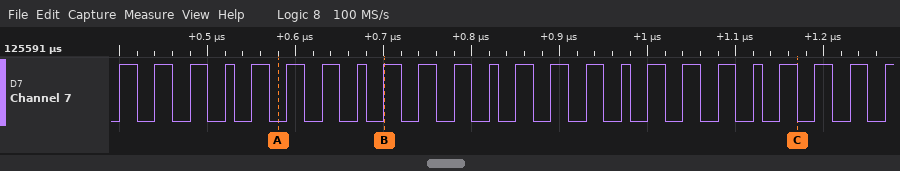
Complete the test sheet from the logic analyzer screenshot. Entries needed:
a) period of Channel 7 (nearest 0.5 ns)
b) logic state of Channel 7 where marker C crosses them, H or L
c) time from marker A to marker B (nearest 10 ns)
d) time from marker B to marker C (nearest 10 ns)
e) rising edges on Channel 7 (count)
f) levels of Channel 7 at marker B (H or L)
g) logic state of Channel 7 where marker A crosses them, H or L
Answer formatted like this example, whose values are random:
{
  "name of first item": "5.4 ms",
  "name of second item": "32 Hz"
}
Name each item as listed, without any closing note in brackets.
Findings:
{
  "period of Channel 7": "38 ns",
  "logic state of Channel 7 where marker C crosses them, H or L": "Channel 7=L",
  "time from marker A to marker B": "120 ns",
  "time from marker B to marker C": "470 ns",
  "rising edges on Channel 7": "24",
  "levels of Channel 7 at marker B": "Channel 7=H",
  "logic state of Channel 7 where marker A crosses them, H or L": "Channel 7=L"
}
